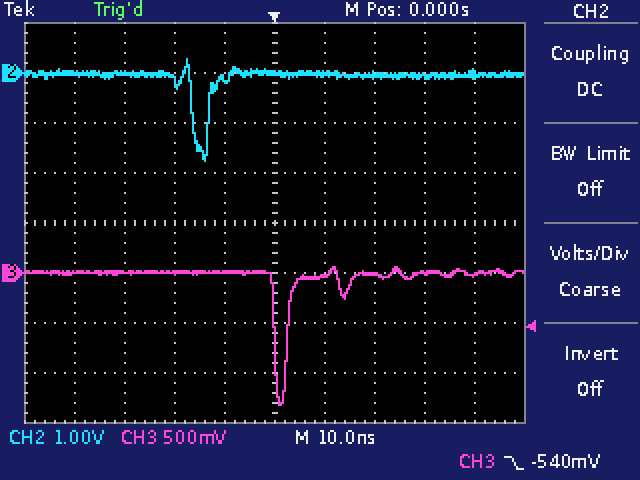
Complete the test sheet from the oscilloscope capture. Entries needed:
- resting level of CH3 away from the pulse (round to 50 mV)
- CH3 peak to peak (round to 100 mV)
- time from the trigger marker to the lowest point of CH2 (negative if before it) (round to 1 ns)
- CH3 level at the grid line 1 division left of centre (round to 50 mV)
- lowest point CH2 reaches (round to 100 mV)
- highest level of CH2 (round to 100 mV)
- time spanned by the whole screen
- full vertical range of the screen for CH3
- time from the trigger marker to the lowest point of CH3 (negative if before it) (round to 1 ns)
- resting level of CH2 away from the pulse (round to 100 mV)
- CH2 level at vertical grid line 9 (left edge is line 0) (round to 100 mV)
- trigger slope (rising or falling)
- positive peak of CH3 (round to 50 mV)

0 mV
1.40 V
-14 ns
0 mV
-1.8 V
300 mV
100 ns
4 V
+1 ns
0.0 V
0.0 V
falling
50 mV
